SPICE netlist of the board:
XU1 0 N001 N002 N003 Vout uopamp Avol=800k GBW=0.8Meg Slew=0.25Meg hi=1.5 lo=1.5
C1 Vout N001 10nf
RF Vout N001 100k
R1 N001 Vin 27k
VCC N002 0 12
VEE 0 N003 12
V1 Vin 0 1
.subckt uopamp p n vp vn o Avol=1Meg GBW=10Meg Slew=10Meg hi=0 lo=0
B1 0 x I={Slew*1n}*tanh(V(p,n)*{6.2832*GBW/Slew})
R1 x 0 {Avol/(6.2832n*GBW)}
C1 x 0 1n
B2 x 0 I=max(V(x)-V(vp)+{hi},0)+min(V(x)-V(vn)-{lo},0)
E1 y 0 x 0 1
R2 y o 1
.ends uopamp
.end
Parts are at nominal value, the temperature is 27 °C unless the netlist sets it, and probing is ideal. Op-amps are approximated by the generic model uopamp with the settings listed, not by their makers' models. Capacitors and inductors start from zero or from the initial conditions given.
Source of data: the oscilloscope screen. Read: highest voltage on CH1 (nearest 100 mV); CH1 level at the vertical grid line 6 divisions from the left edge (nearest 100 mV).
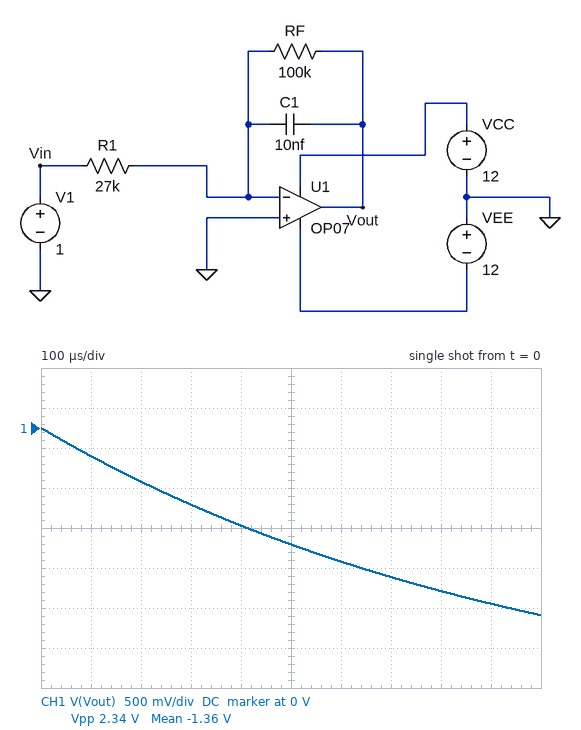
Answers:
0 V
-1.7 V
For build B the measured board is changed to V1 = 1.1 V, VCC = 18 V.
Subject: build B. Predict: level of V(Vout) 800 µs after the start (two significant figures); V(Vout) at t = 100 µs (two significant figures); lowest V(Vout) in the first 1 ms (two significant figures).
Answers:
-2.2 V
-390 mV
-2.6 V
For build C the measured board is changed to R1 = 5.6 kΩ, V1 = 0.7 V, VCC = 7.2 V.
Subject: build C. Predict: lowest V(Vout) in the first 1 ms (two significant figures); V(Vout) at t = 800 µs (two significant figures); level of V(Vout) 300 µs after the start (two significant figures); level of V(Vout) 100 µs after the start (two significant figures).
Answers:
-7.9 V
-6.9 V
-3.2 V
-1.2 V
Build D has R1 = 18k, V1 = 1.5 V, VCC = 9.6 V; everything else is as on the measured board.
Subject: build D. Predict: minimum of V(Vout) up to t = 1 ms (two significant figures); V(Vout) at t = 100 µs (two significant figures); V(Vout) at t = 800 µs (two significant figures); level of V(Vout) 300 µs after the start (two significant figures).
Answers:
-5.3 V
-790 mV
-4.6 V
-2.2 V
